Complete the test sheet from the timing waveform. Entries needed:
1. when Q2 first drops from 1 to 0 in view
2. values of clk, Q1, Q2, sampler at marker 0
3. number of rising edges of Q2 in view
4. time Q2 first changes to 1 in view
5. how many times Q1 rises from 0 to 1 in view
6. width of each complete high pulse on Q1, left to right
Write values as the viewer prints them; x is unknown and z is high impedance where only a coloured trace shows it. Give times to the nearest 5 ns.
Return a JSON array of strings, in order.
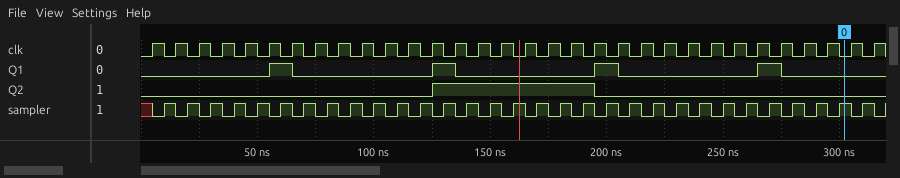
["195 ns", "clk=0, Q1=0, Q2=0, sampler=1", "1", "125 ns", "4", "10 ns, 10 ns, 10 ns, 10 ns"]
